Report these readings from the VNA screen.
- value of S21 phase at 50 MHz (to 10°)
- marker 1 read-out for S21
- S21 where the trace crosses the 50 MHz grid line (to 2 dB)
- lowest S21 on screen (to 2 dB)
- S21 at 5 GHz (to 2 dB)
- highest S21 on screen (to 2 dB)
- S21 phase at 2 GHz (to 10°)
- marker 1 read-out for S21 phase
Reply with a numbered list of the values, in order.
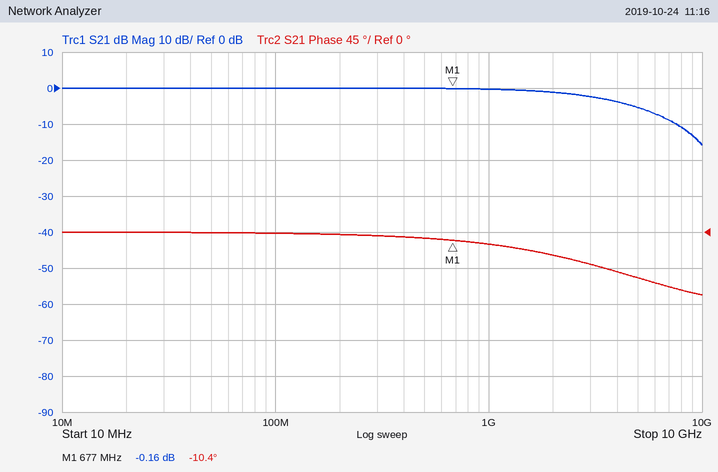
1. 0°
2. -0.16 dB
3. 0 dB
4. -16 dB
5. -6 dB
6. 0 dB
7. -30°
8. -10.4°
